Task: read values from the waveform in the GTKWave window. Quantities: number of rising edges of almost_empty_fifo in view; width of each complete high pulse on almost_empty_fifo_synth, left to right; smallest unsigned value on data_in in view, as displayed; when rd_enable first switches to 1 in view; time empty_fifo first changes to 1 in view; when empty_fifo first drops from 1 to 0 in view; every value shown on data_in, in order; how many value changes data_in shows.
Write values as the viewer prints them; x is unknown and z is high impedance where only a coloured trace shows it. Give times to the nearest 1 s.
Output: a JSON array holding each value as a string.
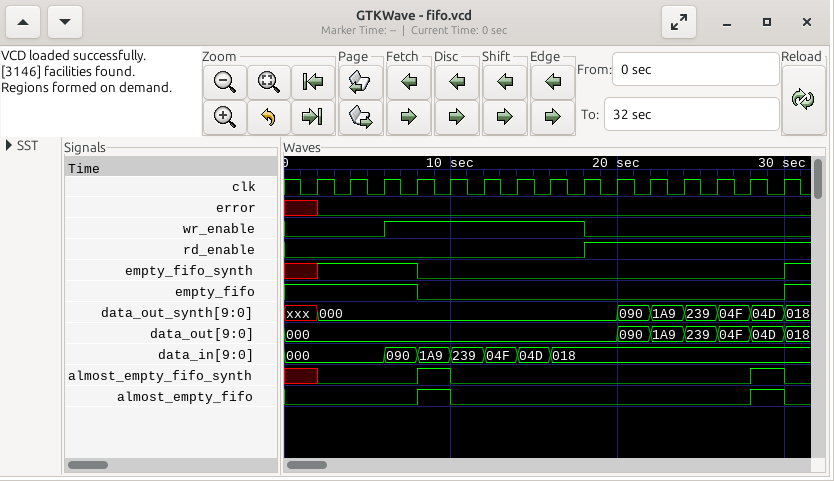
["2", "2 s, 2 s", "000", "18 s", "30 s", "8 s", "000, 090, 1A9, 239, 04F, 04D, 018", "6"]
